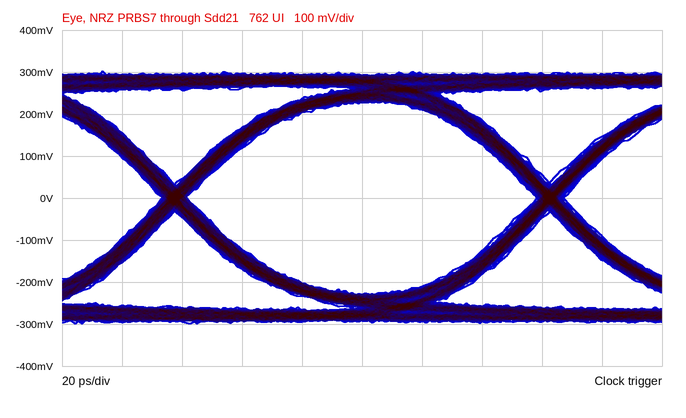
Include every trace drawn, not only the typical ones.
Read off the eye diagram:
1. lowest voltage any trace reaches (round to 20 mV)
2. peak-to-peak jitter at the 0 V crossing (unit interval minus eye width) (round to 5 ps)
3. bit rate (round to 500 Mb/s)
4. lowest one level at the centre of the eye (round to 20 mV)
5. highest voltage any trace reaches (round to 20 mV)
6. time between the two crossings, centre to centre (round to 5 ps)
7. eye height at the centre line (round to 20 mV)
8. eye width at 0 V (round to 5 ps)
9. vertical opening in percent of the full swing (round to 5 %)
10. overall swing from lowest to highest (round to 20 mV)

-300 mV
10 ps
8.0 Gb/s
220 mV
300 mV
125 ps
460 mV
115 ps
75 %
600 mV
